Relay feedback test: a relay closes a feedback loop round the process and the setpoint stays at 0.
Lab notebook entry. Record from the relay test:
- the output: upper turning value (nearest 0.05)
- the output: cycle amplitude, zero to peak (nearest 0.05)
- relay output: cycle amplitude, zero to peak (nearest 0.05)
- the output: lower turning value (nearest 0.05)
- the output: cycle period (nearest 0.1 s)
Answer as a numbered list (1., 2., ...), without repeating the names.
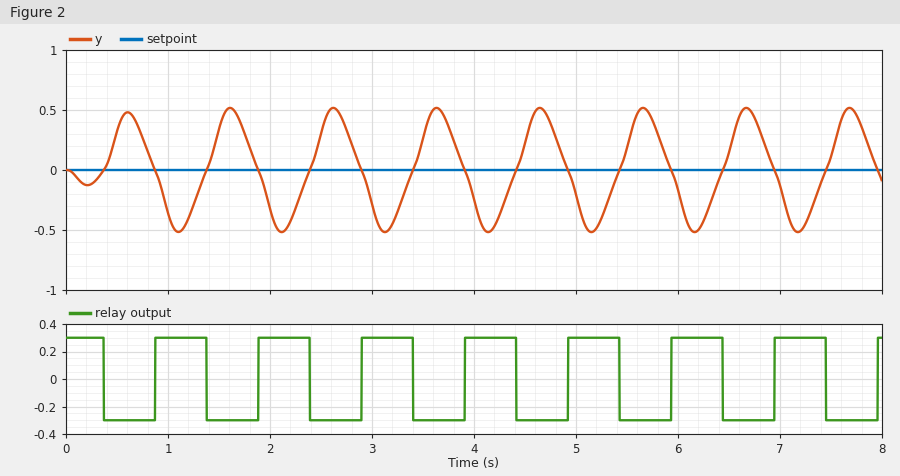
1. 0.50
2. 0.50
3. 0.30
4. -0.50
5. 1.0 s
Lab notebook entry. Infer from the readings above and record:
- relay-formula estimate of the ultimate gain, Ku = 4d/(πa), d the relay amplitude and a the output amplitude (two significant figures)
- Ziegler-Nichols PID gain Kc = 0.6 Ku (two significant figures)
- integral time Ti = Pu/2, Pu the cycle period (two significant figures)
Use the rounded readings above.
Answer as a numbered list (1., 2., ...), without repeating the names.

1. 0.76
2. 0.46
3. 0.50 s
